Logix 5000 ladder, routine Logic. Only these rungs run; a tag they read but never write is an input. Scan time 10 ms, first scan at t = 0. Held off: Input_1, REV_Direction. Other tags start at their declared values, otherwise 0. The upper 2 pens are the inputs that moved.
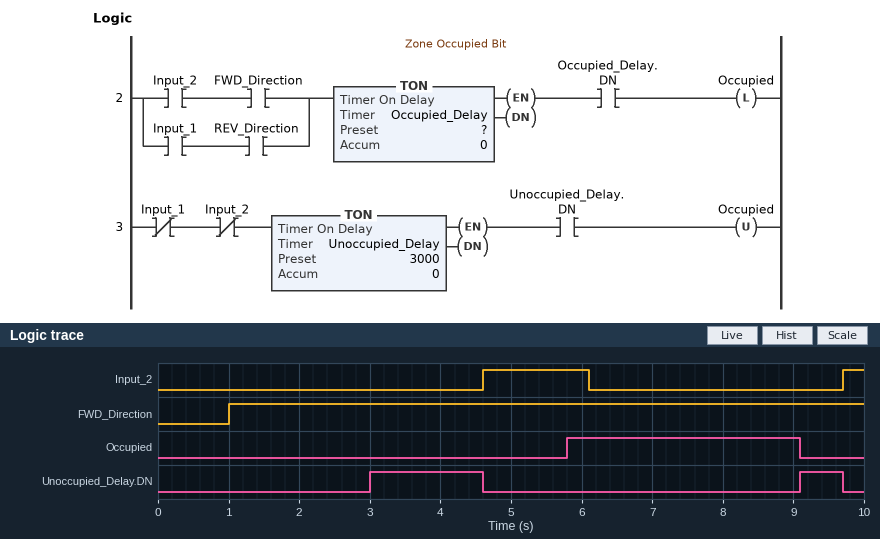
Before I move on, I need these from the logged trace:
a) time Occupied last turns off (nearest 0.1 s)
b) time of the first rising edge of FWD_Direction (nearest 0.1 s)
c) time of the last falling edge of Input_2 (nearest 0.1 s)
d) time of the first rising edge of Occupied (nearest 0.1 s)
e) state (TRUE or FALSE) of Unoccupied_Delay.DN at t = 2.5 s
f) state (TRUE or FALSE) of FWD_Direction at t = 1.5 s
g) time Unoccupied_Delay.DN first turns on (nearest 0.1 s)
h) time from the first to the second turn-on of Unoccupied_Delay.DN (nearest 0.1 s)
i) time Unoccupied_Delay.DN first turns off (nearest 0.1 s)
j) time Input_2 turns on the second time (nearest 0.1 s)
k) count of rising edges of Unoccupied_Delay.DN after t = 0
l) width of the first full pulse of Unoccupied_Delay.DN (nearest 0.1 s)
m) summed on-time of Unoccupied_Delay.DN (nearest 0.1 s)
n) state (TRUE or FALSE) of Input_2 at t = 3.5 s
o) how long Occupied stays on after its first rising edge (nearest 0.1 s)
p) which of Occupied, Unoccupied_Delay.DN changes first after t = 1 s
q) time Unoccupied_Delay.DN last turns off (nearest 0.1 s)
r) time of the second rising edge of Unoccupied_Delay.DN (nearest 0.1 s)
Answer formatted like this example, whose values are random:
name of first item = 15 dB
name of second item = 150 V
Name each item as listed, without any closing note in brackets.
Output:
time Occupied last turns off = 9.1 s
time of the first rising edge of FWD_Direction = 1.0 s
time of the last falling edge of Input_2 = 6.1 s
time of the first rising edge of Occupied = 5.8 s
state (TRUE or FALSE) of Unoccupied_Delay.DN at t = 2.5 s = FALSE
state (TRUE or FALSE) of FWD_Direction at t = 1.5 s = TRUE
time Unoccupied_Delay.DN first turns on = 3.0 s
time from the first to the second turn-on of Unoccupied_Delay.DN = 6.1 s
time Unoccupied_Delay.DN first turns off = 4.6 s
time Input_2 turns on the second time = 9.7 s
count of rising edges of Unoccupied_Delay.DN after t = 0 = 2
width of the first full pulse of Unoccupied_Delay.DN = 1.6 s
summed on-time of Unoccupied_Delay.DN = 2.2 s
state (TRUE or FALSE) of Input_2 at t = 3.5 s = FALSE
how long Occupied stays on after its first rising edge = 3.3 s
which of Occupied, Unoccupied_Delay.DN changes first after t = 1 s = Unoccupied_Delay.DN
time Unoccupied_Delay.DN last turns off = 9.7 s
time of the second rising edge of Unoccupied_Delay.DN = 9.1 s
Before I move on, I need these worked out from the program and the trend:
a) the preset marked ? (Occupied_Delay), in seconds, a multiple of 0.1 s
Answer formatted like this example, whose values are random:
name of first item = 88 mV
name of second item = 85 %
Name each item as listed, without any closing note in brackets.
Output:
the preset marked ? (Occupied_Delay), in seconds, a multiple of 0.1 s = 1.2 s
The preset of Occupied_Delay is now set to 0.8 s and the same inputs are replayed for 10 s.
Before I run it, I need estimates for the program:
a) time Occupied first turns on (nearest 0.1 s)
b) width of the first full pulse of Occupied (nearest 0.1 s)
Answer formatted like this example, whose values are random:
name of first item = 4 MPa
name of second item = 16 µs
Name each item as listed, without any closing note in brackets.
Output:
time Occupied first turns on = 5.4 s
width of the first full pulse of Occupied = 3.7 s
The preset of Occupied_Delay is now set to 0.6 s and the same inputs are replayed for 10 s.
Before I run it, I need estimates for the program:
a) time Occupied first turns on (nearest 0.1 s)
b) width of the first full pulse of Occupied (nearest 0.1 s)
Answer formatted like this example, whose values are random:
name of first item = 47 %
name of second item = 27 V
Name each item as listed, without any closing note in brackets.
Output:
time Occupied first turns on = 5.2 s
width of the first full pulse of Occupied = 3.9 s
